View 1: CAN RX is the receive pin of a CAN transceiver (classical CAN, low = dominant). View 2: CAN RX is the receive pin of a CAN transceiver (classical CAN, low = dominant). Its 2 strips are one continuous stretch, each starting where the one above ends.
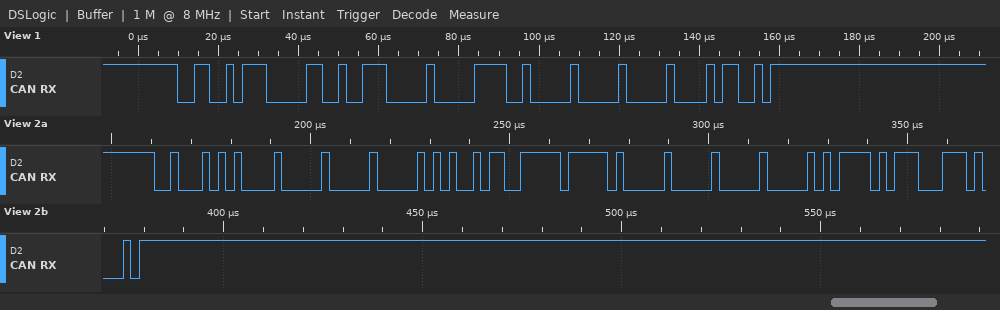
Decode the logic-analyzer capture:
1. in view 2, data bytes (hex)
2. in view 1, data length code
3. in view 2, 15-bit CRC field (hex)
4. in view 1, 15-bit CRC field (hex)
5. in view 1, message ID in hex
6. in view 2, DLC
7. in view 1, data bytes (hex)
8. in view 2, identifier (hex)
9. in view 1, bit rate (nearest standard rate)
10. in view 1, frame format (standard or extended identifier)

00 05 2C FF E0 00 00 BD
4
0x38E8
0x002C
0x32E
8
9C 00 E4 00
0x22A
500 kbit/s
standard
